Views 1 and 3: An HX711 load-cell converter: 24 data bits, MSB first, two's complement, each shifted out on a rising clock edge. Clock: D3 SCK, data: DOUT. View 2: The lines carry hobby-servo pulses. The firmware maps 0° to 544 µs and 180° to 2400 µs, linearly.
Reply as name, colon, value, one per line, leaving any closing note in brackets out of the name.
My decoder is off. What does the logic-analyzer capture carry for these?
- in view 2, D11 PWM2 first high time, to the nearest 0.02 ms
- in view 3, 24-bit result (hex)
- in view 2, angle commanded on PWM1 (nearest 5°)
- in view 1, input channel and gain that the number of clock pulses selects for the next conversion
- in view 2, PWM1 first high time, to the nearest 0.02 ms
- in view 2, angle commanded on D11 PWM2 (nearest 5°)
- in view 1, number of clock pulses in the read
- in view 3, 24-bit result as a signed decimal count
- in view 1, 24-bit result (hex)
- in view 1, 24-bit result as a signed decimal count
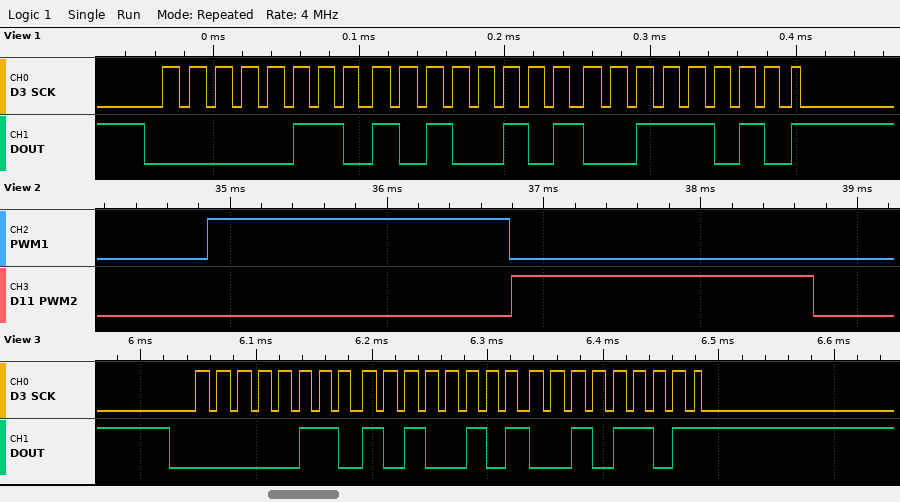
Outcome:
in view 2, D11 PWM2 first high time, to the nearest 0.02 ms: 1.92 ms
in view 3, 24-bit result: 0x06A52D
in view 2, angle commanded on PWM1: 135°
in view 1, input channel and gain that the number of clock pulses selects for the next conversion: channel A, gain 128
in view 2, PWM1 first high time, to the nearest 0.02 ms: 1.92 ms
in view 2, angle commanded on D11 PWM2: 135°
in view 1, number of clock pulses in the read: 25
in view 3, 24-bit result as a signed decimal count: 435501
in view 1, 24-bit result: 0x06A53A
in view 1, 24-bit result as a signed decimal count: 435514
